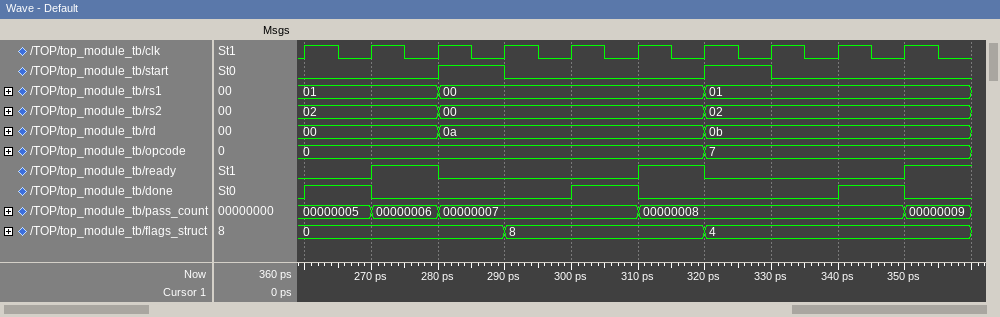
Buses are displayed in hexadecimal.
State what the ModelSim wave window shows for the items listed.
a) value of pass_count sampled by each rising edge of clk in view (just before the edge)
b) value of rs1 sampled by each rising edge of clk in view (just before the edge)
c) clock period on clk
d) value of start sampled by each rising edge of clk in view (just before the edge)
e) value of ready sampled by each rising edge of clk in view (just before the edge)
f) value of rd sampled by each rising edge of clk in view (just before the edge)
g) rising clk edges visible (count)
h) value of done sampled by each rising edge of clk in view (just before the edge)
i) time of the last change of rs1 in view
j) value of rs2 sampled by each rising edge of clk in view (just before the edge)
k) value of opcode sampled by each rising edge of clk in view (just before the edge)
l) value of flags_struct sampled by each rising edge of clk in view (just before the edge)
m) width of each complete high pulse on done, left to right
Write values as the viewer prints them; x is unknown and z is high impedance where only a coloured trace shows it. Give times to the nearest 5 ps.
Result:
00000005, 00000005, 00000006, 00000007, 00000007, 00000007, 00000008, 00000008, 00000008, 00000008
01, 01, 01, 00, 00, 00, 00, 01, 01, 01
10 ps
0 0 0 1 0 0 0 1 0 0
0 0 1 0 0 0 1 0 0 0
00, 00, 00, 0a, 0a, 0a, 0a, 0b, 0b, 0b
10
0 1 0 0 0 1 0 0 0 1
320 ps
02, 02, 02, 00, 00, 00, 00, 02, 02, 02
0, 0, 0, 0, 0, 0, 0, 7, 7, 7
0, 0, 0, 0, 8, 8, 8, 4, 4, 4
10 ps, 10 ps, 10 ps
